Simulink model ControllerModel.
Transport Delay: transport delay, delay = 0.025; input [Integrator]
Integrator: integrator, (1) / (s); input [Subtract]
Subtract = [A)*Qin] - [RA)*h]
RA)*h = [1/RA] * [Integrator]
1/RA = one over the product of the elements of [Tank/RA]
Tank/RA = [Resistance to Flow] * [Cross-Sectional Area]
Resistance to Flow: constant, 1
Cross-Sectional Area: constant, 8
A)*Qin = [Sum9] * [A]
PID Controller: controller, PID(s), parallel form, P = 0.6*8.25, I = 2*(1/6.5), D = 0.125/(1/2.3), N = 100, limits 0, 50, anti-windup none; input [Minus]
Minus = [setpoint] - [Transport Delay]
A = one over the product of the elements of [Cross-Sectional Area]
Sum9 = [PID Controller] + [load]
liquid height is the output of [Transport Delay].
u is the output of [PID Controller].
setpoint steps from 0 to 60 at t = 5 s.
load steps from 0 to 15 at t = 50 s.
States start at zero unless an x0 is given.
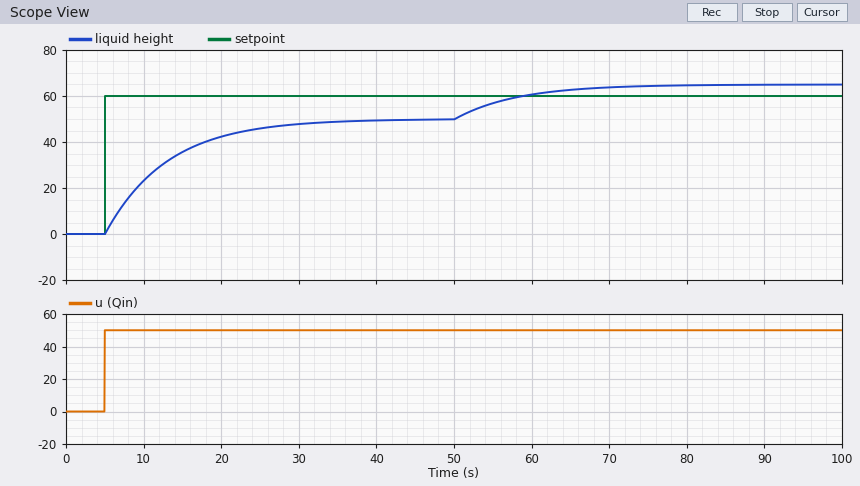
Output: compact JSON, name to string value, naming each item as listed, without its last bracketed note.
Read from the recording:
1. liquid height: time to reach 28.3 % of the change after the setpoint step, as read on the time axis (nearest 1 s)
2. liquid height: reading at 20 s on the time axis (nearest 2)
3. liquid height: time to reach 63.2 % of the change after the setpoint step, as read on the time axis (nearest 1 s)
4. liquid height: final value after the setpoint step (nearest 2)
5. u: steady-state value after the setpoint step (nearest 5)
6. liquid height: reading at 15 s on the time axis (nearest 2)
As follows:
{"liquid height: time to reach 28.3 % of the change after the setpoint step, as read on the time axis": "8 s", "liquid height: reading at 20 s on the time axis": "42", "liquid height: time to reach 63.2 % of the change after the setpoint step, as read on the time axis": "13 s", "liquid height: final value after the setpoint step": "50", "u: steady-state value after the setpoint step": "50", "liquid height: reading at 15 s on the time axis": "36"}
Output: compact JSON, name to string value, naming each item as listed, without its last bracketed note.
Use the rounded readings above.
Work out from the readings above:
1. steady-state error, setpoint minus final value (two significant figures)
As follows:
{"steady-state error, setpoint minus final value": "10"}
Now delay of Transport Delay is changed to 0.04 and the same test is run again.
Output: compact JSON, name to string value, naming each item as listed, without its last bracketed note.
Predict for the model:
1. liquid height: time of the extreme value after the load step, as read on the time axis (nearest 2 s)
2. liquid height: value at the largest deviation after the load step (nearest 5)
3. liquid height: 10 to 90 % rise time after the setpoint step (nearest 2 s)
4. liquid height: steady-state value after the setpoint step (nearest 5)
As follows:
{"liquid height: time of the extreme value after the load step, as read on the time axis": "100 s", "liquid height: value at the largest deviation after the load step": "65", "liquid height: 10 to 90 % rise time after the setpoint step": "18 s", "liquid height: steady-state value after the setpoint step": "50"}
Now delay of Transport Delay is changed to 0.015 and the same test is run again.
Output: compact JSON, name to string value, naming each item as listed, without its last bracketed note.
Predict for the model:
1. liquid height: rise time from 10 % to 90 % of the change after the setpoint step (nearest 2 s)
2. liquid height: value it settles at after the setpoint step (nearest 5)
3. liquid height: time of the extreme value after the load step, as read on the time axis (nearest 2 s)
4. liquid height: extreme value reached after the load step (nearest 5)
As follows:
{"liquid height: rise time from 10 % to 90 % of the change after the setpoint step": "18 s", "liquid height: value it settles at after the setpoint step": "50", "liquid height: time of the extreme value after the load step, as read on the time axis": "100 s", "liquid height: extreme value reached after the load step": "65"}
